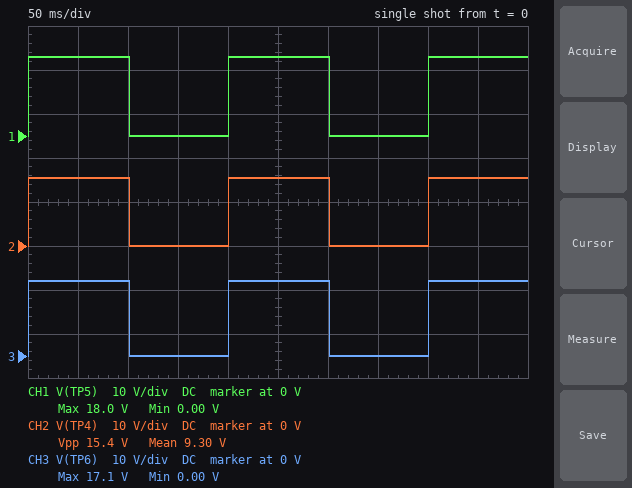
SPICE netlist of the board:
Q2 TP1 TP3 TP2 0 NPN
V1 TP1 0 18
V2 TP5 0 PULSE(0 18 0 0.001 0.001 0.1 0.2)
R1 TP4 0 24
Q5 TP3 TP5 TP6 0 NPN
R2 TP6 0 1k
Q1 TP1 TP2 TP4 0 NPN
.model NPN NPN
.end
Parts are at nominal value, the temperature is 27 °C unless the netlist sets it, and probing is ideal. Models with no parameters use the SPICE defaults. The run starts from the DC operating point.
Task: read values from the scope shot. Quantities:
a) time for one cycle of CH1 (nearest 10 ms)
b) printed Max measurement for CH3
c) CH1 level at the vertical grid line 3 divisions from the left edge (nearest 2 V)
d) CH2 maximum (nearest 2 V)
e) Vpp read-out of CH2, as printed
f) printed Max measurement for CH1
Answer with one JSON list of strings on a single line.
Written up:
["200 ms", "17.1 V", "0 V", "16 V", "15.4 V", "18.0 V"]
